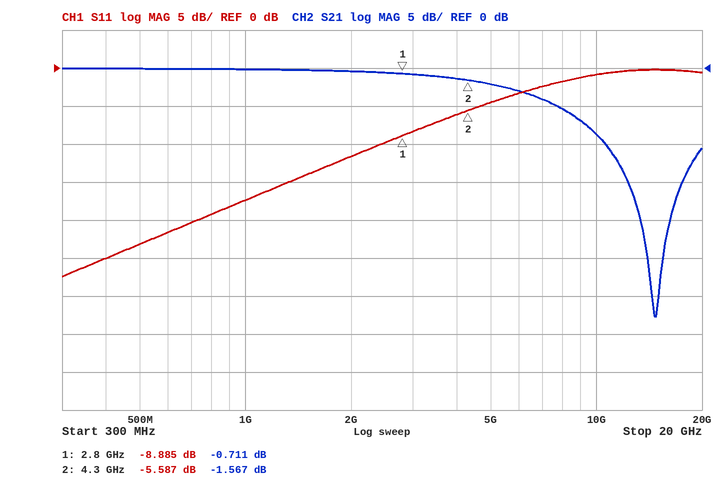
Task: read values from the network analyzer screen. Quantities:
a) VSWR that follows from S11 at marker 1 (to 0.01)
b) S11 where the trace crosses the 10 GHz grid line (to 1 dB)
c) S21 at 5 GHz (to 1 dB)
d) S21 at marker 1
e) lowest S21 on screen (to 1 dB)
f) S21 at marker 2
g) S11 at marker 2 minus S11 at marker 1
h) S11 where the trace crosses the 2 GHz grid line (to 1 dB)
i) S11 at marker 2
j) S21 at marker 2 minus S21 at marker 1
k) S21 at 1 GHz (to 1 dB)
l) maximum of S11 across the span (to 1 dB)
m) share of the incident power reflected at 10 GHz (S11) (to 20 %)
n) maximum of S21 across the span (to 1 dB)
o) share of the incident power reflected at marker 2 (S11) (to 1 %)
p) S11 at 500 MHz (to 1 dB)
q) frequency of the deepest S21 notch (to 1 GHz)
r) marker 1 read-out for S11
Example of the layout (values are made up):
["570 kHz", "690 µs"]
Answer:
["2.12", "-1 dB", "-2 dB", "-0.711 dB", "-33 dB", "-1.567 dB", "3.298 dB", "-12 dB", "-5.587 dB", "-0.856 dB", "0 dB", "0 dB", "80 %", "0 dB", "28 %", "-23 dB", "15 GHz", "-8.885 dB"]
